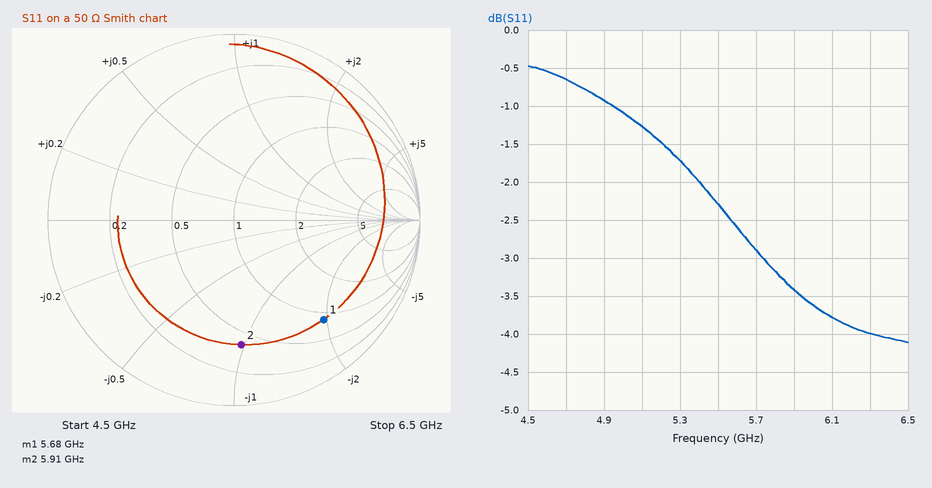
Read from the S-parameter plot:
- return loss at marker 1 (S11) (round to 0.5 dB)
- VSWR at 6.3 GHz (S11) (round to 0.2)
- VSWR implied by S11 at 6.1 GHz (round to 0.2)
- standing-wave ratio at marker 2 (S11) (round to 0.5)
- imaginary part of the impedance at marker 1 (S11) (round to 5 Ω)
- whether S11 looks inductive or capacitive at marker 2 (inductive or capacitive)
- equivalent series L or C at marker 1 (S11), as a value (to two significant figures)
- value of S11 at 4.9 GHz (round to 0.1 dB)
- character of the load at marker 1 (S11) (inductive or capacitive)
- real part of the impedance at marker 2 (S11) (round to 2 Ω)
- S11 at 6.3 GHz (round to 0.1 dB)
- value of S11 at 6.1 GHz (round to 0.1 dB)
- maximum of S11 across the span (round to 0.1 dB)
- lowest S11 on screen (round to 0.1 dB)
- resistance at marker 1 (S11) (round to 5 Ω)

3.0 dB
4.4
4.6
5.0
-95 Ω
capacitive
290 fF
-0.9 dB
capacitive
20 Ω
-4.0 dB
-3.8 dB
-0.5 dB
-4.1 dB
45 Ω
